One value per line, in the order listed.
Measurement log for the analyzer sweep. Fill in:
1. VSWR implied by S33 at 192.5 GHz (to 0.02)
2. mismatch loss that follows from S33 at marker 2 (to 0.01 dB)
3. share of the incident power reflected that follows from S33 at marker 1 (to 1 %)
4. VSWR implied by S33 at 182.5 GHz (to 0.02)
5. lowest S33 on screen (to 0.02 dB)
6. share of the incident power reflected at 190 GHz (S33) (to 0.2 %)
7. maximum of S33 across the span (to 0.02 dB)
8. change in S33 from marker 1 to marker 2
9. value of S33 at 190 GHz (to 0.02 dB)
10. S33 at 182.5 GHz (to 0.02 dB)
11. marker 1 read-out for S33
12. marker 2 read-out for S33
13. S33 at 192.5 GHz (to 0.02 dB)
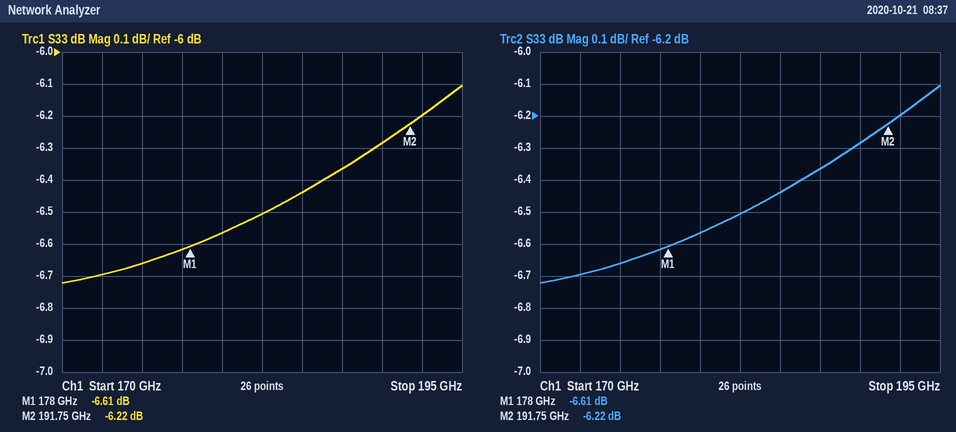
2.92
1.18 dB
22 %
2.80
-6.72 dB
23.6 %
-6.10 dB
0.39 dB
-6.28 dB
-6.50 dB
-6.61 dB
-6.22 dB
-6.20 dB
